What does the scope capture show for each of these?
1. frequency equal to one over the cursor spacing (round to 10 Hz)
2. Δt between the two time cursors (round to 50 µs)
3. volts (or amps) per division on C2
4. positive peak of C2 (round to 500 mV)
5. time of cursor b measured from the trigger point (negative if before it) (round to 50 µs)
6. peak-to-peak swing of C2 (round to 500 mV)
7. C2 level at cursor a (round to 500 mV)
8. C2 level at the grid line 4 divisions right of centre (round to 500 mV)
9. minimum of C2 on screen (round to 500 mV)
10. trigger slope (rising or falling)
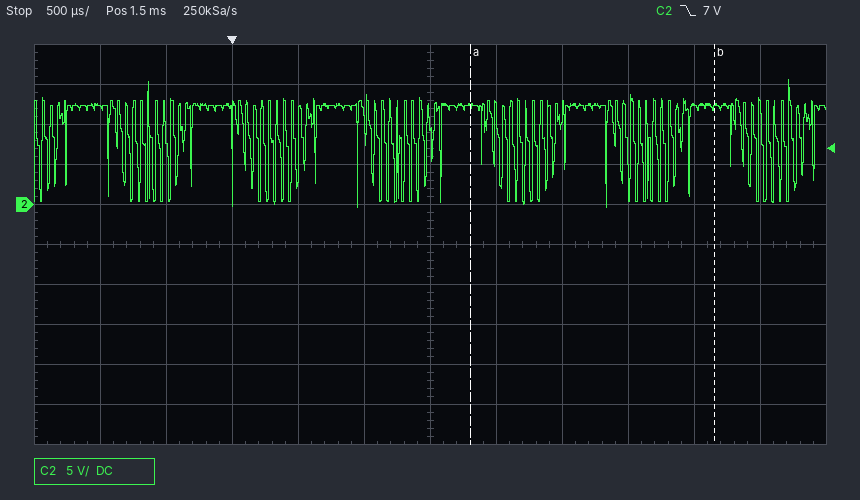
540 Hz
1.85 ms
5 V
15.5 V
+3.65 ms
16.0 V
12.5 V
12.5 V
-500 mV
falling
